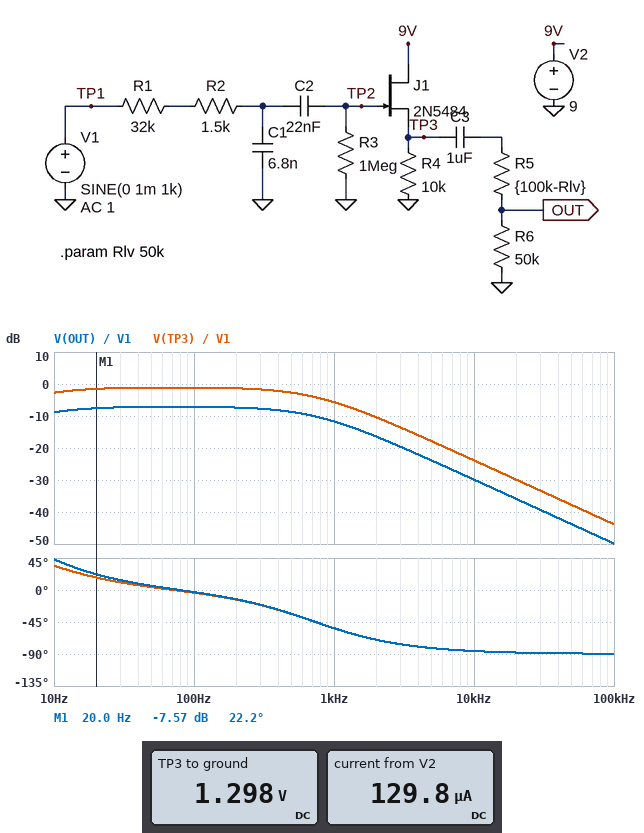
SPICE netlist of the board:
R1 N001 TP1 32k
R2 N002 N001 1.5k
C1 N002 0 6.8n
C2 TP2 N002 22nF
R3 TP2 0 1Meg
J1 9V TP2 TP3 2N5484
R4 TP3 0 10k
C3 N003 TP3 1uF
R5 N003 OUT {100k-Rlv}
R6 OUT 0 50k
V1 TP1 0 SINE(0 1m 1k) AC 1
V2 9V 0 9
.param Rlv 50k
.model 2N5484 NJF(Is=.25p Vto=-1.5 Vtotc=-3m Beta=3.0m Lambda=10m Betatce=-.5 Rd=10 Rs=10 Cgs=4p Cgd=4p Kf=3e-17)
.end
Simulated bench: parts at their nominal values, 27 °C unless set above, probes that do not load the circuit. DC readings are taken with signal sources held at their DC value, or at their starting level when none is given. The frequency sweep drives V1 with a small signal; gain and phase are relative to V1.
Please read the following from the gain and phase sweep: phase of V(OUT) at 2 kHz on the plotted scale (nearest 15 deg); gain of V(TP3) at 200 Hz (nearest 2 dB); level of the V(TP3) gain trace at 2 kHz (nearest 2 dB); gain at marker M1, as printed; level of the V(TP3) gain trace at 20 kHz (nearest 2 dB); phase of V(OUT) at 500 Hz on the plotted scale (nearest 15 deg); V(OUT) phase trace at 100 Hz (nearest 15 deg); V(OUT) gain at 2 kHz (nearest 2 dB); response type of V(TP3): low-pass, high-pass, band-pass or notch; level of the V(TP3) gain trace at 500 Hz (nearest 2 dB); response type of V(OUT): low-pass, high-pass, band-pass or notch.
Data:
-75 deg
-2 dB
-10 dB
-7.57 dB
-30 dB
-30 deg
0 deg
-16 dB
low-pass
-2 dB
low-pass
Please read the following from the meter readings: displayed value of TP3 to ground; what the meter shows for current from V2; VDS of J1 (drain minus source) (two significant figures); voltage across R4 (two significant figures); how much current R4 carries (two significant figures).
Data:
1.298 V
129.8 µA
7.7 V
1.3 V
130 µA
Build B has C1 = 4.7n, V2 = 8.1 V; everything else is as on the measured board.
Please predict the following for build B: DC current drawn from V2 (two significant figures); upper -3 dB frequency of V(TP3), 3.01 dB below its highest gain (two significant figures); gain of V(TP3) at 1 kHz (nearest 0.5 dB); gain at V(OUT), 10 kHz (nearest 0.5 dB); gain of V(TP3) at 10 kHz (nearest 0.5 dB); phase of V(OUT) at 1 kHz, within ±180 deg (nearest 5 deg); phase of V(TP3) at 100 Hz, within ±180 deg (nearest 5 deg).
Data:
130 µA
1.1 kHz
-4.0 dB
-26.5 dB
-20.5 dB
-45 deg
0 deg
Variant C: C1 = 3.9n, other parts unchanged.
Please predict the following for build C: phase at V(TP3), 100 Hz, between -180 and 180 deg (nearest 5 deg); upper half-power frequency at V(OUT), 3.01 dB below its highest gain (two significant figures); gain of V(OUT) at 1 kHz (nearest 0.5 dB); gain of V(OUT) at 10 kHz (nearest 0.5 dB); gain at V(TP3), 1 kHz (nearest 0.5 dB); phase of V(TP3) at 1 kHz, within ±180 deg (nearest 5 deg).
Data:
0 deg
1.3 kHz
-9.0 dB
-25.0 dB
-3.0 dB
-40 deg
